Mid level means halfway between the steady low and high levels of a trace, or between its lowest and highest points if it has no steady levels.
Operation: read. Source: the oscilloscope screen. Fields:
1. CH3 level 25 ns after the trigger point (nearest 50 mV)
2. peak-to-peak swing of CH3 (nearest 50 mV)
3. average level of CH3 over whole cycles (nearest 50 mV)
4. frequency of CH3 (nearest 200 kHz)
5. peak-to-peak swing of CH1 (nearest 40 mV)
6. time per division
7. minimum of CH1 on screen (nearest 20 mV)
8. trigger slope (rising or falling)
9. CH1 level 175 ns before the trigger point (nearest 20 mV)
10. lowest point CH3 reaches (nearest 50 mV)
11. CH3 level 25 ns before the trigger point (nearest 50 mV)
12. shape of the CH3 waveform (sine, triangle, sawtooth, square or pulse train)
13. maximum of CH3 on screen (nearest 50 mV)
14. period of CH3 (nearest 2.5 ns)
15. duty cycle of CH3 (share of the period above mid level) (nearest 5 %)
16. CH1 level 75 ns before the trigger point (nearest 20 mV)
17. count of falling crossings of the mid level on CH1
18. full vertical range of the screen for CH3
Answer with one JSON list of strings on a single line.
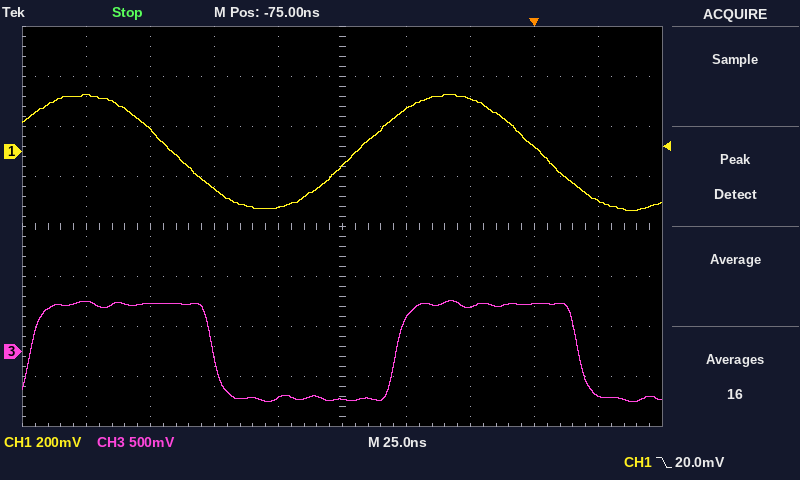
["-450 mV", "1.00 V", "0 mV", "7.0 MHz", "480 mV", "25 ns", "-240 mV", "falling", "220 mV", "-500 mV", "450 mV", "square", "500 mV", "142.5 ns", "50 %", "-60 mV", "2", "4 V"]
